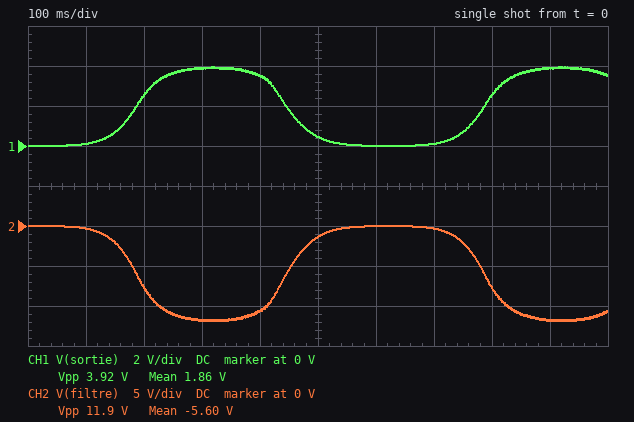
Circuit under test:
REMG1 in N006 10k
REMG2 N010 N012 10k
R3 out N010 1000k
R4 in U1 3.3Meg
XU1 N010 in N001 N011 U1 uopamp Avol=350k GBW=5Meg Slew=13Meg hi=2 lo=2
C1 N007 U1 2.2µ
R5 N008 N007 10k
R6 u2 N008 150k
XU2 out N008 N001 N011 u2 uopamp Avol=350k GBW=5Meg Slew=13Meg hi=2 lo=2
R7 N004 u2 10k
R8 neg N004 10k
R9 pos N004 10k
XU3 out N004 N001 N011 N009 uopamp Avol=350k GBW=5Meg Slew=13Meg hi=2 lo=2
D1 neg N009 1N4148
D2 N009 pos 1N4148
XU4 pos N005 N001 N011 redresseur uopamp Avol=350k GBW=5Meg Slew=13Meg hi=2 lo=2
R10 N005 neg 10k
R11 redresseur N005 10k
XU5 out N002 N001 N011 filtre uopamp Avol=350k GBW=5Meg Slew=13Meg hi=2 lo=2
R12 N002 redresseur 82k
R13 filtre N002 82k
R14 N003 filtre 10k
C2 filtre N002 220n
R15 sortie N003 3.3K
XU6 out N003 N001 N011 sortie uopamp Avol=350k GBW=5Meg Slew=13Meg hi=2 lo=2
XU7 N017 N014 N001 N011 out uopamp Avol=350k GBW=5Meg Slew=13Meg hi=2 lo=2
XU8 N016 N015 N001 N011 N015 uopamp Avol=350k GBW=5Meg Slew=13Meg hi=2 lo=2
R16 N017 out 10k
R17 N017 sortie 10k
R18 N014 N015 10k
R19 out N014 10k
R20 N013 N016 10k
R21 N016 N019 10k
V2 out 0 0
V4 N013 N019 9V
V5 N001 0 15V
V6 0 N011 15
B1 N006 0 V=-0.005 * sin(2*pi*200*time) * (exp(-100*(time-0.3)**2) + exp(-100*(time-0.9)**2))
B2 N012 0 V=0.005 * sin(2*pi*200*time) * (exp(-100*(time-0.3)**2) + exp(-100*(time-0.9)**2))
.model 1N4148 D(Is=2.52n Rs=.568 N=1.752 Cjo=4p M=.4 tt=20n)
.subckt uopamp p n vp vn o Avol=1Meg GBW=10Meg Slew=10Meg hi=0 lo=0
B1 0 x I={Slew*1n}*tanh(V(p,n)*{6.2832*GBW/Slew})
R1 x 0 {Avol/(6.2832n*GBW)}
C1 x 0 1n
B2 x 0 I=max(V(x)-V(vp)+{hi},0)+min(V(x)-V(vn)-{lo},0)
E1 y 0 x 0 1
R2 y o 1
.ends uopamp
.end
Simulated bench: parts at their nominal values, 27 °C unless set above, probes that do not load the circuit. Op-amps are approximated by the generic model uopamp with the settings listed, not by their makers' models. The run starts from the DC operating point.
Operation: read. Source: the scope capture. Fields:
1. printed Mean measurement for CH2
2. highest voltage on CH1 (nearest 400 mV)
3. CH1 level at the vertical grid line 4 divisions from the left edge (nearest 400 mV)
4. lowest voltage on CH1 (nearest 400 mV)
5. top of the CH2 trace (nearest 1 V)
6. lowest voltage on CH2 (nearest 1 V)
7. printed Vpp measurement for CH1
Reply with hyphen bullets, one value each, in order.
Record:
- -5.60 V
- 4.0 V
- 3.6 V
- 0 V
- 0 V
- -12 V
- 3.92 V
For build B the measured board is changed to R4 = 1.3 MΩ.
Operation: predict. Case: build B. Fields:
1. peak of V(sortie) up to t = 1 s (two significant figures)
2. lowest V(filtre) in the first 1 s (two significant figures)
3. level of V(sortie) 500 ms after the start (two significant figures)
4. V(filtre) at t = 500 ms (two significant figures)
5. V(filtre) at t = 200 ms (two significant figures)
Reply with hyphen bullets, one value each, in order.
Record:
- 3.3 V
- -10 V
- 180 mV
- -550 mV
- -3.2 V
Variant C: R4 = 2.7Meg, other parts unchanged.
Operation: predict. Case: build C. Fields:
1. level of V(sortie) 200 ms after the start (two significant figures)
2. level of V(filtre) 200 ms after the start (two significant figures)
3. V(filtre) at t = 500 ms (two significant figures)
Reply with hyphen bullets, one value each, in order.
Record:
- 2.2 V
- -6.6 V
- -1.1 V
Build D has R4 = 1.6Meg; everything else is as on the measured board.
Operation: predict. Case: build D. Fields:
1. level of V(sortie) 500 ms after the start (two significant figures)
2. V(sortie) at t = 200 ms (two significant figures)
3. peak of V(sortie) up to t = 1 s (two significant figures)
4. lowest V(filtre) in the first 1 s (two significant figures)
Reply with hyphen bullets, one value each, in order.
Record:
- 220 mV
- 1.3 V
- 3.5 V
- -11 V
